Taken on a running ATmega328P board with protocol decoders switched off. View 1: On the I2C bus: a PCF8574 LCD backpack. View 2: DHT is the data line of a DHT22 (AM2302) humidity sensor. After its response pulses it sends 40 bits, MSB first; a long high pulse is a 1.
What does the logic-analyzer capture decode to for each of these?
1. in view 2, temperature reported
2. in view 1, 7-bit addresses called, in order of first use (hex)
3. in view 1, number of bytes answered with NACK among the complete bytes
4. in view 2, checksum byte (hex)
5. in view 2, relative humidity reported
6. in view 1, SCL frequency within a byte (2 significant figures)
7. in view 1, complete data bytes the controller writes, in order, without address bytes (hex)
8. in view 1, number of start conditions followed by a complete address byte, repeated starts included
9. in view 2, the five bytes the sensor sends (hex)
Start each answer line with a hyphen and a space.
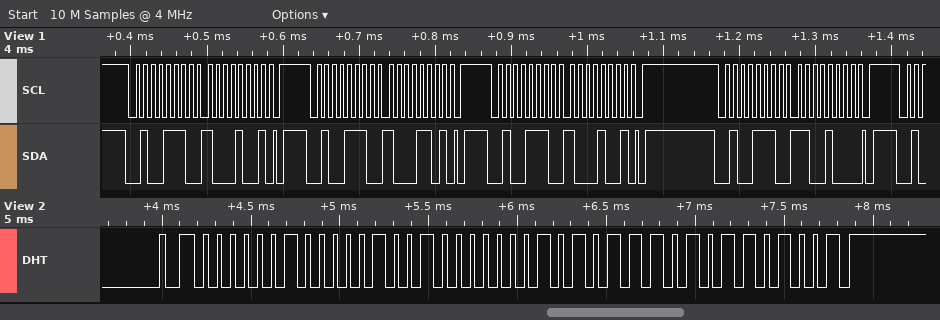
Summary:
- 34.9 °C
- 0x27
- 0
- 0x69
- 52.1 %
- 100 kHz
- 89 8D 89 C8
- 4
- 02 09 01 5D 69
